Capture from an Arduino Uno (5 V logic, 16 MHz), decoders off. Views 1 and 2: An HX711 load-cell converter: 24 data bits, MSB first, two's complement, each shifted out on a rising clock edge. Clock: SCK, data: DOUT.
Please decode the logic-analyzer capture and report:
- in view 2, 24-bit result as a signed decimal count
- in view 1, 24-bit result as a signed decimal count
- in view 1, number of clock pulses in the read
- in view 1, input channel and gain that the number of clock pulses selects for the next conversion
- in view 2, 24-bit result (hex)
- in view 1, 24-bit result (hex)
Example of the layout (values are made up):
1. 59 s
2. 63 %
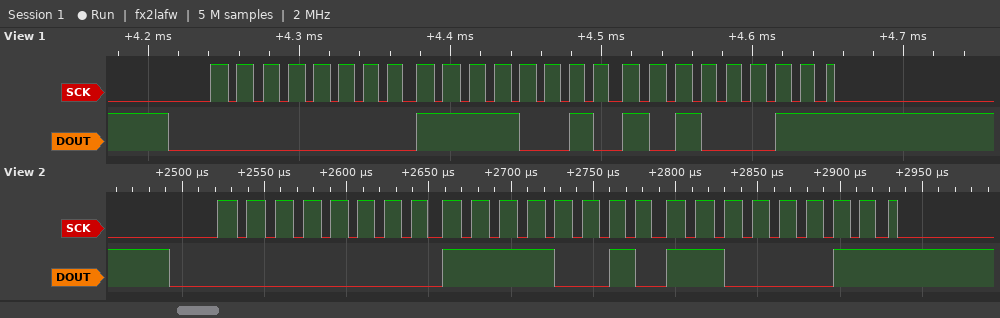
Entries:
1. 62147
2. 62115
3. 25
4. channel A, gain 128
5. 0x00F2C3
6. 0x00F2A3
